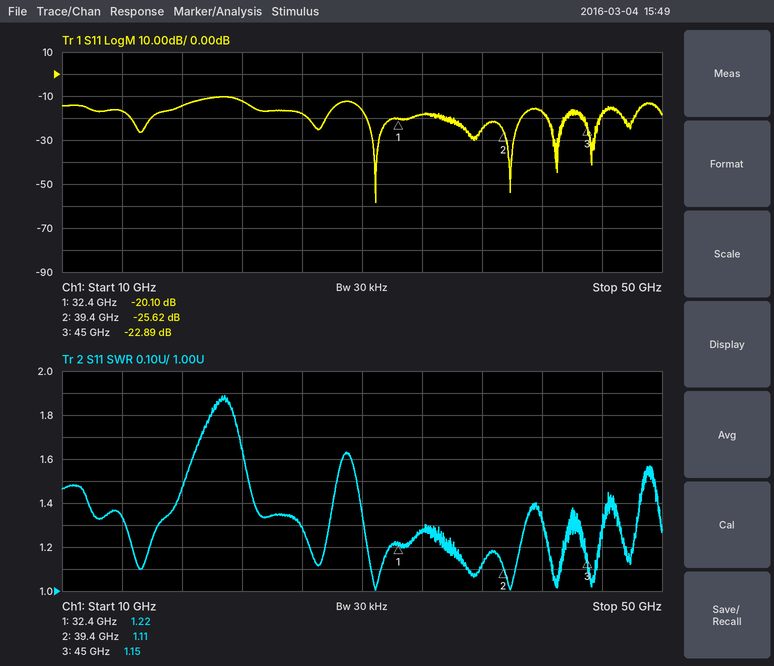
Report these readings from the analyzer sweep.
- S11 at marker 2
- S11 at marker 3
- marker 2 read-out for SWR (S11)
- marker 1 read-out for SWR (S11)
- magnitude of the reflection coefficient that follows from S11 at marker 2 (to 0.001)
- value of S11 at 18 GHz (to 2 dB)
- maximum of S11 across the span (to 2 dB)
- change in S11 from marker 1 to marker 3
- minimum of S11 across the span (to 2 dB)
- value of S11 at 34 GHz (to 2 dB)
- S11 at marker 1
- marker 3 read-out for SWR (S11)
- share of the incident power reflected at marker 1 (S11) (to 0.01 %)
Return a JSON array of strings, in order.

["-25.62 dB", "-22.89 dB", "1.11", "1.22", "0.052", "-14 dB", "-10 dB", "-2.79 dB", "-58 dB", "-18 dB", "-20.10 dB", "1.15", "0.98 %"]
